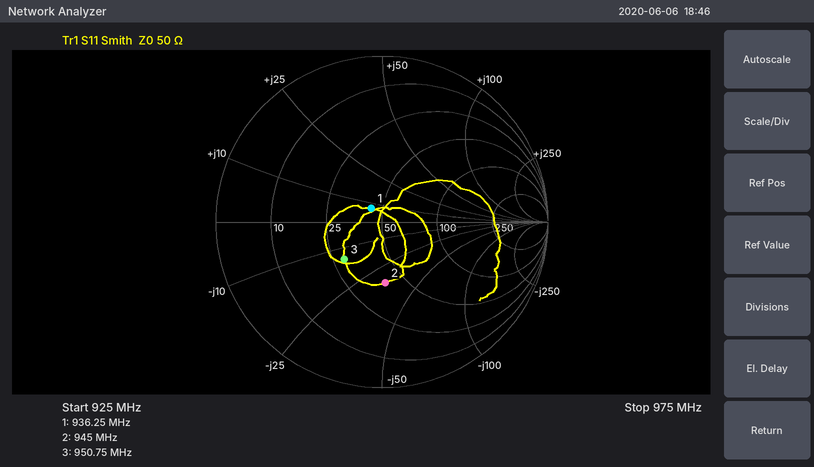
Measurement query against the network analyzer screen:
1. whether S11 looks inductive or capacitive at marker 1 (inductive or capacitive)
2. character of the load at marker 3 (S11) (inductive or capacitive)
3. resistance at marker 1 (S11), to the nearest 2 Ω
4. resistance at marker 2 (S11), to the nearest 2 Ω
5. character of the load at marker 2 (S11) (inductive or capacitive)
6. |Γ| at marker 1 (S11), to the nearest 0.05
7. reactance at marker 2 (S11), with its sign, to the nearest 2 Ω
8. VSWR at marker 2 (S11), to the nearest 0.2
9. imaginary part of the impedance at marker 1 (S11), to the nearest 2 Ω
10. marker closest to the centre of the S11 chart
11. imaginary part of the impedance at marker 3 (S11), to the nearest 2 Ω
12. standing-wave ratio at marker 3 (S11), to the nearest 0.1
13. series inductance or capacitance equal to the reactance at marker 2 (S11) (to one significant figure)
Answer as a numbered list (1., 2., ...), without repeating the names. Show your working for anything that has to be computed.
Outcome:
1. inductive
2. capacitive
3. 44 Ω
4. 40 Ω
5. capacitive
6. 0.10
7. -34 Ω
8. 2.2
9. +8 Ω
10. marker 1
11. -14 Ω
12. 1.9
13. C = 1/(2π × 945 MHz × 34 Ω) ≈ 5 pF
